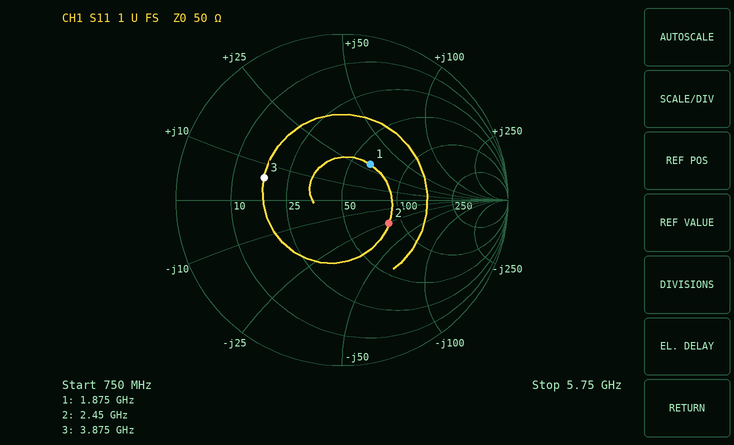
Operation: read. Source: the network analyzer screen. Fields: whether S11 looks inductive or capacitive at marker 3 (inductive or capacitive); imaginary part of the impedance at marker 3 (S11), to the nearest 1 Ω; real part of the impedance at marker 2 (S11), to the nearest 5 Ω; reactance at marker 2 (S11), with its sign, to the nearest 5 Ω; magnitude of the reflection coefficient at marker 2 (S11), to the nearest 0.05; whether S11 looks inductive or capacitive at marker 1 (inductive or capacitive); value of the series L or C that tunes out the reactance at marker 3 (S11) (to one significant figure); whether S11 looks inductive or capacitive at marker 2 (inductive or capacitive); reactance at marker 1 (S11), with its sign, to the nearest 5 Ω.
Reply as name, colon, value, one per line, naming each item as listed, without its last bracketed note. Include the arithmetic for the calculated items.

whether S11 looks inductive or capacitive at marker 3: inductive
imaginary part of the impedance at marker 3 (S11), to the nearest 1 Ω: +6 Ω
real part of the impedance at marker 2 (S11), to the nearest 5 Ω: 85 Ω
reactance at marker 2 (S11), with its sign, to the nearest 5 Ω: -25 Ω
magnitude of the reflection coefficient at marker 2 (S11), to the nearest 0.05: 0.30
whether S11 looks inductive or capacitive at marker 1: inductive
value of the series L or C that tunes out the reactance at marker 3 (S11): C = 1/(2π × 3.875 GHz × 6 Ω) ≈ 7 pF
whether S11 looks inductive or capacitive at marker 2: capacitive
reactance at marker 1 (S11), with its sign, to the nearest 5 Ω: +30 Ω
